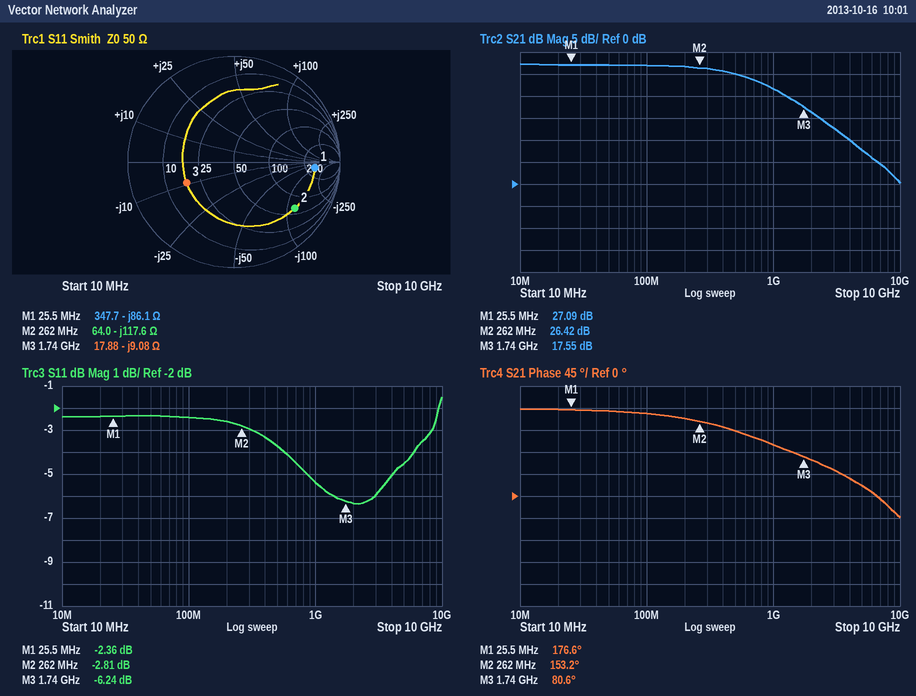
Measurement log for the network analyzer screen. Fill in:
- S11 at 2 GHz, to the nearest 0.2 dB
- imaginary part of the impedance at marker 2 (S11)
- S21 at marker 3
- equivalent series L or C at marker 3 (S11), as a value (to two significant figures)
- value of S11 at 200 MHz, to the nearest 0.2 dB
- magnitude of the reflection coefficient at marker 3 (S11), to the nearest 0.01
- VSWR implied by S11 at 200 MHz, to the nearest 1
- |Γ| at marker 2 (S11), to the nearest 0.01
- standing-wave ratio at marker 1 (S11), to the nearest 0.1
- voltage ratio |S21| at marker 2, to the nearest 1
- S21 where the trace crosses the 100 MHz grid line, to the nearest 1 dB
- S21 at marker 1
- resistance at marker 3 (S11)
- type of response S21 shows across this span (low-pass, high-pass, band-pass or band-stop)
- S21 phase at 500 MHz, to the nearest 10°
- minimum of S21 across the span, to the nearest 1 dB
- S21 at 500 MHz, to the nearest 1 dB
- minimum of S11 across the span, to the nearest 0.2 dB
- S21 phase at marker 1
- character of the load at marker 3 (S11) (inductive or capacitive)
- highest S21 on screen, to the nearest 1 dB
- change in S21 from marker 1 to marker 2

-6.4 dB
-117.6 Ω
17.55 dB
10 pF
-2.6 dB
0.49
7
0.72
7.4
21
27 dB
27.09 dB
17.88 Ω
low-pass
130°
0 dB
25 dB
-6.4 dB
176.6°
capacitive
27 dB
-0.67 dB
